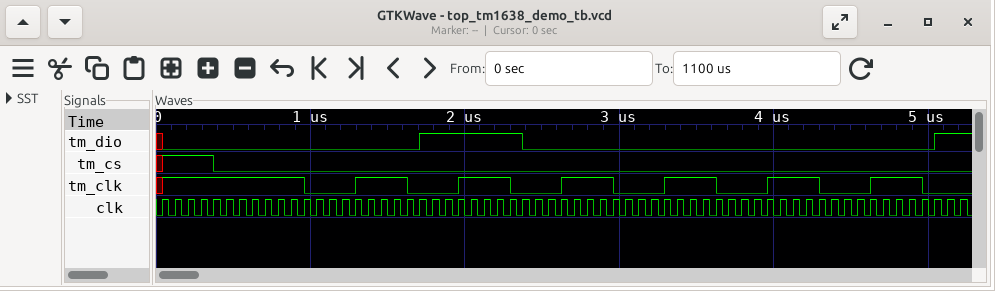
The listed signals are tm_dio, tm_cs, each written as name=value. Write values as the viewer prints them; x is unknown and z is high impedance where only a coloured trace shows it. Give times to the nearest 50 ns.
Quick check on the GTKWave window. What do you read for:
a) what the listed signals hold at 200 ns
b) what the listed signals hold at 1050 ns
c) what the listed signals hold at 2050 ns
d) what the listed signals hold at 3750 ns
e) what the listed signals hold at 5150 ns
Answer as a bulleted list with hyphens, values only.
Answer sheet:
- tm_dio=0, tm_cs=1
- tm_dio=0, tm_cs=0
- tm_dio=1, tm_cs=0
- tm_dio=0, tm_cs=0
- tm_dio=1, tm_cs=0
